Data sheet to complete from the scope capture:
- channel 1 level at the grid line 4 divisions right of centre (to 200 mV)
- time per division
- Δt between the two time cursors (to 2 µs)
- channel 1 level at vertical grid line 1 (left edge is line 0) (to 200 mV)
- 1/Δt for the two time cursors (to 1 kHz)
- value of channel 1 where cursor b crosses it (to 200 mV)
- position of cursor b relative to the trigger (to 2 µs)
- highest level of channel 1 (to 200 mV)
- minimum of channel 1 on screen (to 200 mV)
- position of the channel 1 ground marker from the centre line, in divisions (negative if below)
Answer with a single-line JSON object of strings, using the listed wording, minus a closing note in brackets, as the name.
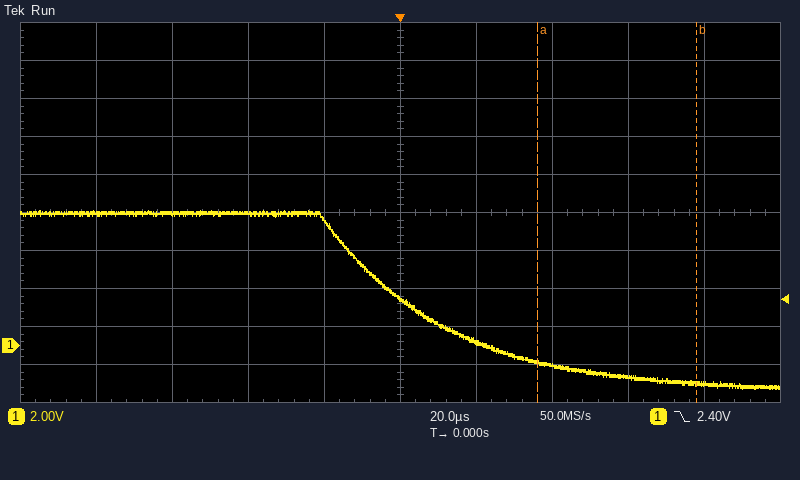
{"channel 1 level at the grid line 4 divisions right of centre": "-2.0 V", "time per division": "20 µs", "Δt between the two time cursors": "42 µs", "channel 1 level at vertical grid line 1 (left edge is line 0)": "7.0 V", "1/Δt for the two time cursors": "24 kHz", "value of channel 1 where cursor b crosses it": "-2.0 V", "position of cursor b relative to the trigger": "+78 µs", "highest level of channel 1": "7.2 V", "minimum of channel 1 on screen": "-2.4 V", "position of the channel 1 ground marker from the centre line, in divisions": "-3.5 div"}
